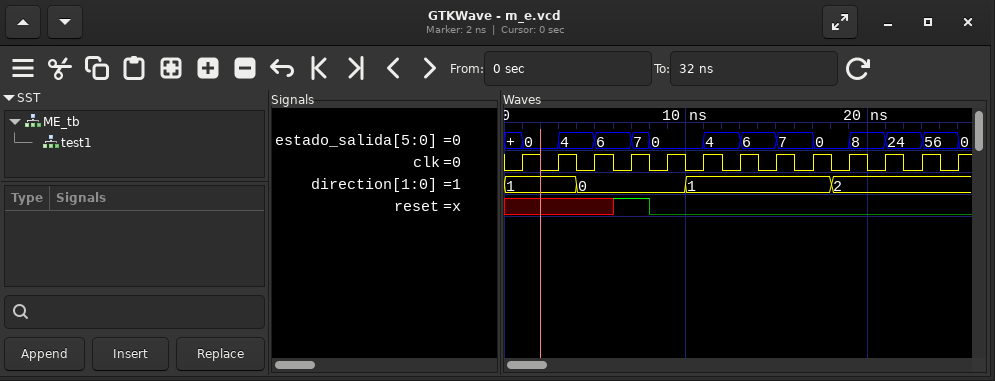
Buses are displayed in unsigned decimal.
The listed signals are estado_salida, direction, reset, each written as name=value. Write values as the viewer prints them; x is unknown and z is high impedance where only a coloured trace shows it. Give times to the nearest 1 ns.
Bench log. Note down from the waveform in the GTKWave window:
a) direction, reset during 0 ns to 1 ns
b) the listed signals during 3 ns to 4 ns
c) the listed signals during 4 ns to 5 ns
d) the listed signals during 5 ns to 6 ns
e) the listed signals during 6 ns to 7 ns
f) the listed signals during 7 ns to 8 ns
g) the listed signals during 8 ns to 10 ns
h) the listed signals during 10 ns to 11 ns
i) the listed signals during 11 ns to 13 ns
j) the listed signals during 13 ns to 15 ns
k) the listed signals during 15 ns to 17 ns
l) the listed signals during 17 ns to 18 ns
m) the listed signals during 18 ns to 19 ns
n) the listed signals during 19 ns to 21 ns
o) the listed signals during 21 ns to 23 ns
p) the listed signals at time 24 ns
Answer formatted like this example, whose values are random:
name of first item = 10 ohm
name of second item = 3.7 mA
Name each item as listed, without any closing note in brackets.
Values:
direction, reset during 0 ns to 1 ns = direction=1, reset=x
the listed signals during 3 ns to 4 ns = estado_salida=4, direction=1, reset=x
the listed signals during 4 ns to 5 ns = estado_salida=4, direction=0, reset=x
the listed signals during 5 ns to 6 ns = estado_salida=6, direction=0, reset=x
the listed signals during 6 ns to 7 ns = estado_salida=6, direction=0, reset=1
the listed signals during 7 ns to 8 ns = estado_salida=7, direction=0, reset=1
the listed signals during 8 ns to 10 ns = estado_salida=0, direction=0, reset=0
the listed signals during 10 ns to 11 ns = estado_salida=0, direction=1, reset=0
the listed signals during 11 ns to 13 ns = estado_salida=4, direction=1, reset=0
the listed signals during 13 ns to 15 ns = estado_salida=6, direction=1, reset=0
the listed signals during 15 ns to 17 ns = estado_salida=7, direction=1, reset=0
the listed signals during 17 ns to 18 ns = estado_salida=0, direction=1, reset=0
the listed signals during 18 ns to 19 ns = estado_salida=0, direction=2, reset=0
the listed signals during 19 ns to 21 ns = estado_salida=8, direction=2, reset=0
the listed signals during 21 ns to 23 ns = estado_salida=24, direction=2, reset=0
the listed signals at time 24 ns = estado_salida=56, direction=2, reset=0
